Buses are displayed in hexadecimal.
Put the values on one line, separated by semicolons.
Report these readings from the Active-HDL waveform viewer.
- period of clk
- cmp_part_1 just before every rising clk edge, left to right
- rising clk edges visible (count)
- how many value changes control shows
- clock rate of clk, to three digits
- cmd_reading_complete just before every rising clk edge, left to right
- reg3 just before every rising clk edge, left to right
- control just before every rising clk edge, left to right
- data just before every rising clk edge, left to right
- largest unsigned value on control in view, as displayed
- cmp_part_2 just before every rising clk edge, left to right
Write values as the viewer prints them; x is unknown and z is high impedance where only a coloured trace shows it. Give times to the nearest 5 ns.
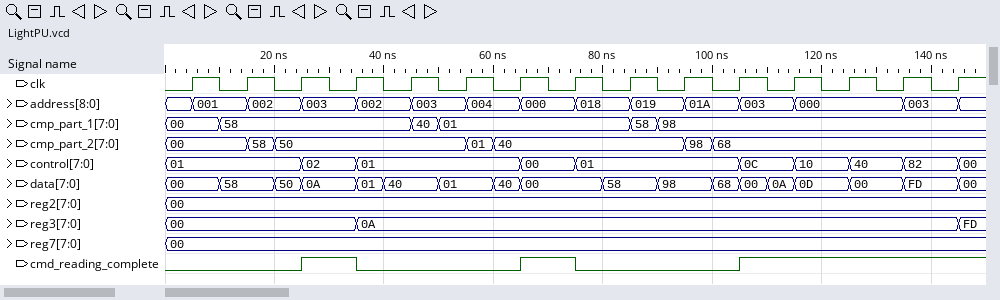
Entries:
10 ns; 00, 58, 58, 58, 58, 01, 01, 01, 01, 98, 98, 98, 98, 98, 98; 15; 9; 100 MHz; 0 0 0 1 0 0 0 1 0 0 0 1 1 1 1; 00, 00, 00, 00, 0A, 0A, 0A, 0A, 0A, 0A, 0A, 0A, 0A, 0A, 0A; 01, 01, 01, 02, 01, 01, 01, 00, 01, 01, 01, 0C, 10, 40, 82; 00, 58, 50, 0A, 40, 01, 40, 00, 58, 98, 68, 0A, 0D, 00, FD; 82; 00, 00, 50, 50, 50, 50, 40, 40, 40, 40, 68, 68, 68, 68, 68
